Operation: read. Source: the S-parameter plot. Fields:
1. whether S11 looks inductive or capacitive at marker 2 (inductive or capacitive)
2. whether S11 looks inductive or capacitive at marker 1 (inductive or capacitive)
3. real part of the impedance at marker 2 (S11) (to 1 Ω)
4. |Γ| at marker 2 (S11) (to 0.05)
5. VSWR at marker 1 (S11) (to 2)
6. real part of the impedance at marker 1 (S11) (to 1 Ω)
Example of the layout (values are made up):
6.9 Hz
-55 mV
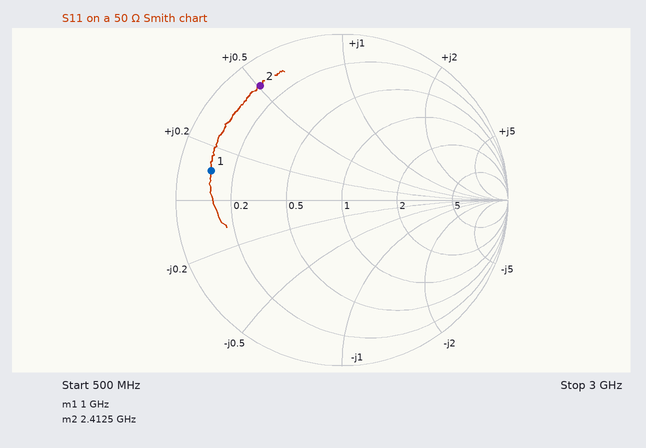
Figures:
inductive
inductive
5 Ω
0.85
10
5 Ω
